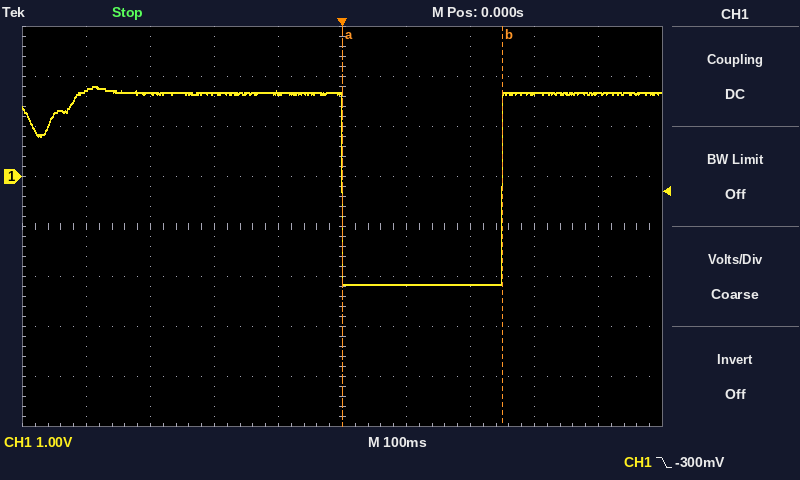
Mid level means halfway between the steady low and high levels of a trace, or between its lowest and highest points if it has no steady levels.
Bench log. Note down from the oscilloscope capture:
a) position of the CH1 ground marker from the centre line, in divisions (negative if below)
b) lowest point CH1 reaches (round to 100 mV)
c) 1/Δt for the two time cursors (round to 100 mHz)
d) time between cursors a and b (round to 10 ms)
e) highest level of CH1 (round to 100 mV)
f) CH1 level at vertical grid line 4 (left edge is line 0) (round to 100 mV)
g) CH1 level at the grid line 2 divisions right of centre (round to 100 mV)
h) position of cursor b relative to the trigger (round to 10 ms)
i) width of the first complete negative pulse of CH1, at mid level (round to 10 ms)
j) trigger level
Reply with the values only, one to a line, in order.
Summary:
+1.0 div
-2.2 V
4.0 Hz
250 ms
1.8 V
1.7 V
-2.2 V
+250 ms
250 ms
-300 mV
